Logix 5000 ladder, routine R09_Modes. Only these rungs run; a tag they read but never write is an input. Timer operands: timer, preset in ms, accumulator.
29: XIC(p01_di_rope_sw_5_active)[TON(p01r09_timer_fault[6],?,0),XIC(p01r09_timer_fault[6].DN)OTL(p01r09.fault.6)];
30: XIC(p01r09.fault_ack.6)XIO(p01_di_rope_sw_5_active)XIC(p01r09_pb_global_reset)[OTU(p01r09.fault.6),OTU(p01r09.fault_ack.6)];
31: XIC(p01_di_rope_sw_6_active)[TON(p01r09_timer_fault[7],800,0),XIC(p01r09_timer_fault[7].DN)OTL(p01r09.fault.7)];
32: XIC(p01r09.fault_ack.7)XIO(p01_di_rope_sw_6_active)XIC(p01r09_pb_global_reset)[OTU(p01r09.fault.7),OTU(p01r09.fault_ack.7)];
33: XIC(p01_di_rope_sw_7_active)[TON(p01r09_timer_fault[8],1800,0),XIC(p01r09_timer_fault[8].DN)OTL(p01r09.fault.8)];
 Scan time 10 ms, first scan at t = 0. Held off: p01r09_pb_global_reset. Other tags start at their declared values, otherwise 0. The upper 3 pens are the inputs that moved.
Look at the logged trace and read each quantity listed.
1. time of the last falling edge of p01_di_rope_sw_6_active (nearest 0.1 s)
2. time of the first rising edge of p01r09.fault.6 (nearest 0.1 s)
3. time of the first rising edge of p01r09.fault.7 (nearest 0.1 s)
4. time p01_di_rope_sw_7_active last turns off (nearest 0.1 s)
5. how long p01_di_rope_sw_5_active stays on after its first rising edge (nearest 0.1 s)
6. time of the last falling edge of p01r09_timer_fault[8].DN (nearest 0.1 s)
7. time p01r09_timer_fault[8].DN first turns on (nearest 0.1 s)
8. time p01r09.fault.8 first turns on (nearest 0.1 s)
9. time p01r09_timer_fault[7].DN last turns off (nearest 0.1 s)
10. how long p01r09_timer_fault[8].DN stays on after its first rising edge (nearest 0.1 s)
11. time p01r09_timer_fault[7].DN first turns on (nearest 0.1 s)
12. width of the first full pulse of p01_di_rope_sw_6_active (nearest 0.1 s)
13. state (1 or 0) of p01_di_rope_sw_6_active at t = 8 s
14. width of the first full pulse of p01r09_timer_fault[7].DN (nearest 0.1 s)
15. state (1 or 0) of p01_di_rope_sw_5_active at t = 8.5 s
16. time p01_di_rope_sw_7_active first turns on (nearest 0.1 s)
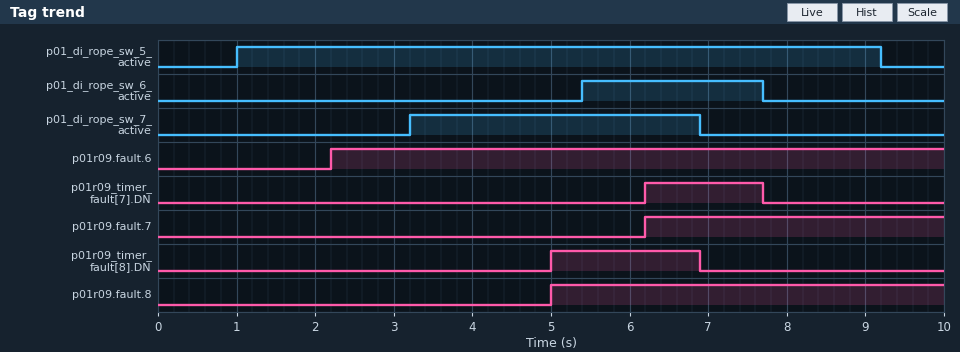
7.7 s
2.2 s
6.2 s
6.9 s
8.2 s
6.9 s
5.0 s
5.0 s
7.7 s
1.9 s
6.2 s
2.3 s
0
1.5 s
1
3.2 s
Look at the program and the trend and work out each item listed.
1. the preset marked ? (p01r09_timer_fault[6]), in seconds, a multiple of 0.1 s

1.2 s
